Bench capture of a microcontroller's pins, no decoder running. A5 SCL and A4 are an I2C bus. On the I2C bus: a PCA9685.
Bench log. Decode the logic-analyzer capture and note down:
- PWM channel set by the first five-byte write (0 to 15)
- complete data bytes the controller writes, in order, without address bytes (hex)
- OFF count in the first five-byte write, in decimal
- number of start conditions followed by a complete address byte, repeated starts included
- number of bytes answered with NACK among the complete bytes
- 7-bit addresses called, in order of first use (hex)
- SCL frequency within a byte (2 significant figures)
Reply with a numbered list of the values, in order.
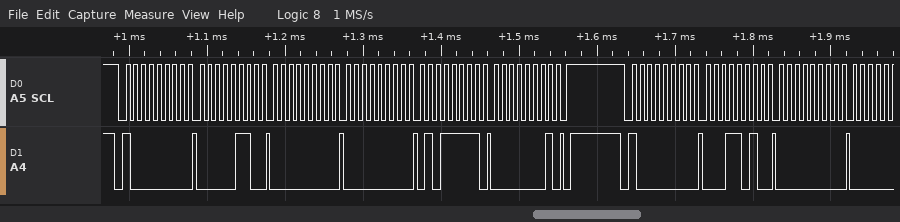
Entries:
1. 0
2. 06 00 00 5F 01 1A 00
3. 351
4. 2
5. 0
6. 0x40
7. 100 kHz
